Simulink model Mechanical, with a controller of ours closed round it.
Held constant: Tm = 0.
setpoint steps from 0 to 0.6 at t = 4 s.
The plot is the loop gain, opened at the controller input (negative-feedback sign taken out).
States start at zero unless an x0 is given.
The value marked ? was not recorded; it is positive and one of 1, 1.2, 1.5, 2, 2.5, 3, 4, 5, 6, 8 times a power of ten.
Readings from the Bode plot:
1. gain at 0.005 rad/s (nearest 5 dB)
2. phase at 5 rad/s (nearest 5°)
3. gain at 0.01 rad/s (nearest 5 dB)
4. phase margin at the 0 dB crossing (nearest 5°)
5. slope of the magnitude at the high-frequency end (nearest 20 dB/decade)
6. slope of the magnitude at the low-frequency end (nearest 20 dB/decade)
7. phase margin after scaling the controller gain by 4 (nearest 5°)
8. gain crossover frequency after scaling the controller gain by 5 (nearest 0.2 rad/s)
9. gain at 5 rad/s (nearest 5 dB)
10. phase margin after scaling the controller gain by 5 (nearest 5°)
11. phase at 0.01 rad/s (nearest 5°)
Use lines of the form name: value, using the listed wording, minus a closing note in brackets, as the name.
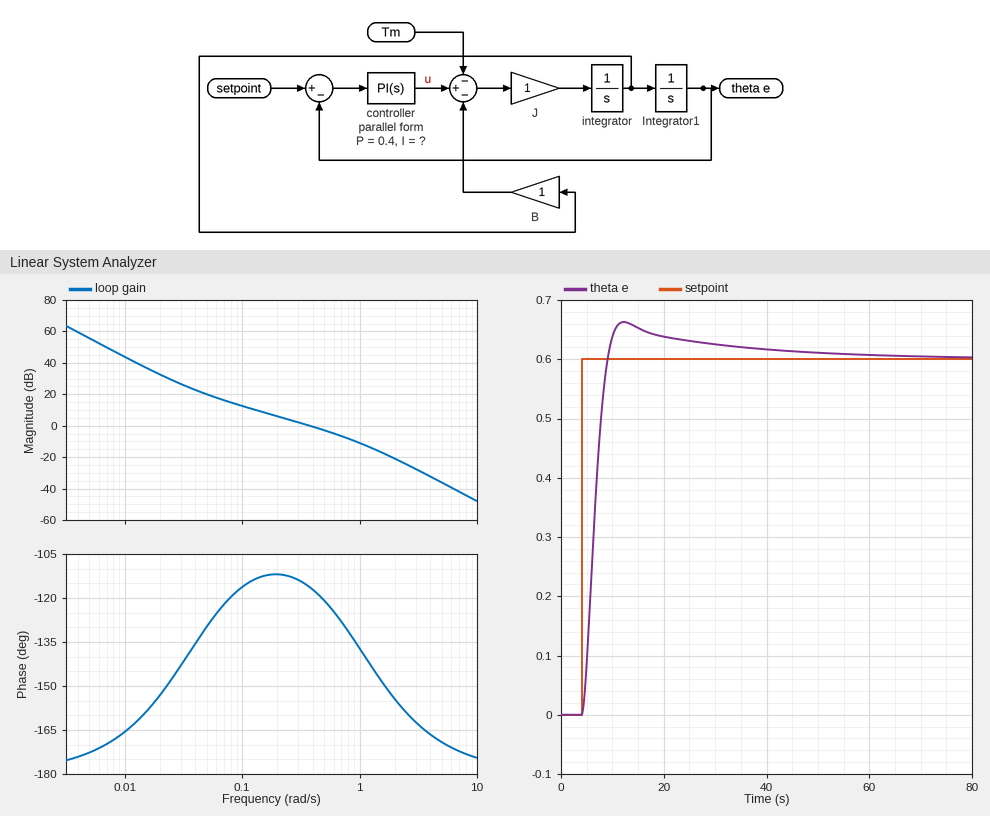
gain at 0.005 rad/s: 55 dB
phase at 5 rad/s: -170°
gain at 0.01 rad/s: 45 dB
phase margin at the 0 dB crossing: 65°
slope of the magnitude at the high-frequency end: -40 dB/decade
slope of the magnitude at the low-frequency end: -40 dB/decade
phase margin after scaling the controller gain by 4: 40°
gain crossover frequency after scaling the controller gain by 5: 1.2 rad/s
gain at 5 rad/s: -35 dB
phase margin after scaling the controller gain by 5: 35°
phase at 0.01 rad/s: -165°
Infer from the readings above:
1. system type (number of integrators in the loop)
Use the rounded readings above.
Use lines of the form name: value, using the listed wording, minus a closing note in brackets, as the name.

system type: 2
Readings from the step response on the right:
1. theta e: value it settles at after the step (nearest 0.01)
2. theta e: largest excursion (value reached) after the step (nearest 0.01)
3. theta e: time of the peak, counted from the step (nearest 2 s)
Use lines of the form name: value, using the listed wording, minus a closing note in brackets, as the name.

theta e: value it settles at after the step: 0.60
theta e: largest excursion (value reached) after the step: 0.66
theta e: time of the peak, counted from the step: 8 s
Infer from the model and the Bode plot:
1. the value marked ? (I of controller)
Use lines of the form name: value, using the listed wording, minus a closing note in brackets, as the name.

the value marked ?: 0.015
